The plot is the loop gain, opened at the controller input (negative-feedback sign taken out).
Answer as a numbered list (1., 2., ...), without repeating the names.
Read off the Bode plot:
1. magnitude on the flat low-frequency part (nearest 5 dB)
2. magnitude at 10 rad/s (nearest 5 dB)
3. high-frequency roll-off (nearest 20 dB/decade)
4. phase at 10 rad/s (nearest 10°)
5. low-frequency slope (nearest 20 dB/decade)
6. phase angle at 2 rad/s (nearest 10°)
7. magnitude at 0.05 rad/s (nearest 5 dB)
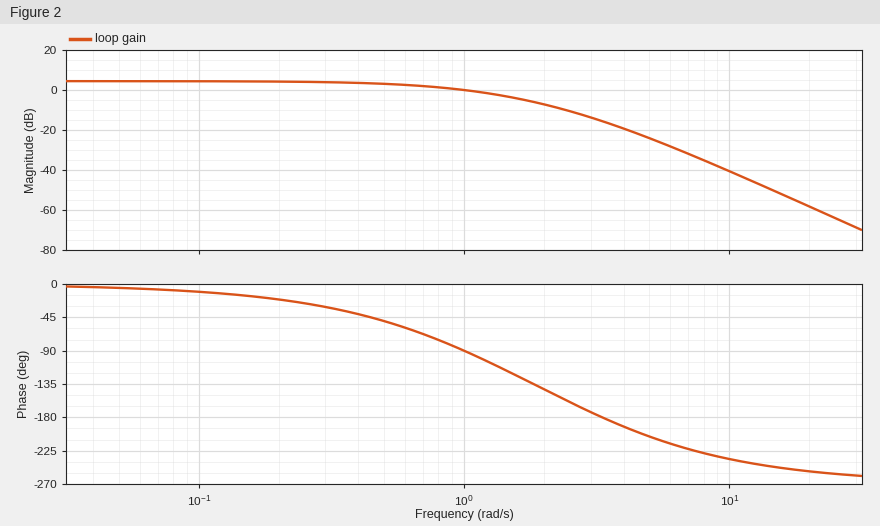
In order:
1. 5 dB
2. -40 dB
3. -60 dB/decade
4. -240°
5. 0 dB/decade
6. -140°
7. 5 dB
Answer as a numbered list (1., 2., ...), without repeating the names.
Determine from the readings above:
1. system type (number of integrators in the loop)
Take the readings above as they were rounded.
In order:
1. 0
